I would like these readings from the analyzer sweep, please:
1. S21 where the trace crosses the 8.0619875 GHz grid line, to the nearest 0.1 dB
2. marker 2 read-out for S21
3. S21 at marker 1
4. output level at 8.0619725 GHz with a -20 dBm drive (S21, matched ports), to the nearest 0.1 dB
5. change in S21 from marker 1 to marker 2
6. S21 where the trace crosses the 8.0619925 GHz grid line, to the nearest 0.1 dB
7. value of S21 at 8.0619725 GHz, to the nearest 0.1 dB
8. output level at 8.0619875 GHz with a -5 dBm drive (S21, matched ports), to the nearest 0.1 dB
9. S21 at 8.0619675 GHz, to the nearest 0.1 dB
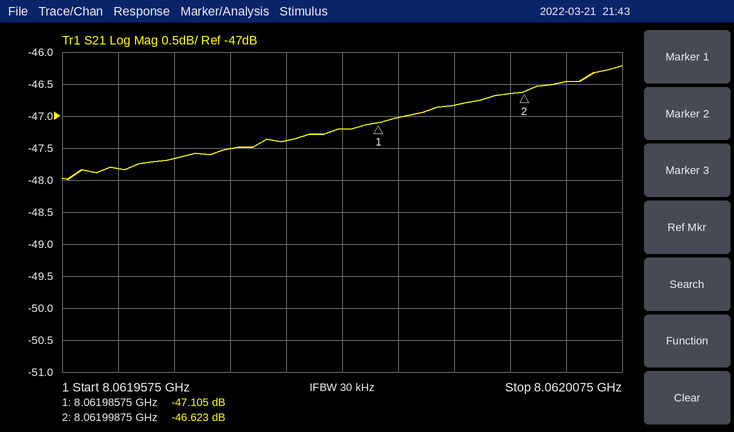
-47.0 dB
-46.623 dB
-47.105 dB
-67.5 dBm
0.482 dB
-46.8 dB
-47.5 dB
-52.0 dBm
-47.7 dB
